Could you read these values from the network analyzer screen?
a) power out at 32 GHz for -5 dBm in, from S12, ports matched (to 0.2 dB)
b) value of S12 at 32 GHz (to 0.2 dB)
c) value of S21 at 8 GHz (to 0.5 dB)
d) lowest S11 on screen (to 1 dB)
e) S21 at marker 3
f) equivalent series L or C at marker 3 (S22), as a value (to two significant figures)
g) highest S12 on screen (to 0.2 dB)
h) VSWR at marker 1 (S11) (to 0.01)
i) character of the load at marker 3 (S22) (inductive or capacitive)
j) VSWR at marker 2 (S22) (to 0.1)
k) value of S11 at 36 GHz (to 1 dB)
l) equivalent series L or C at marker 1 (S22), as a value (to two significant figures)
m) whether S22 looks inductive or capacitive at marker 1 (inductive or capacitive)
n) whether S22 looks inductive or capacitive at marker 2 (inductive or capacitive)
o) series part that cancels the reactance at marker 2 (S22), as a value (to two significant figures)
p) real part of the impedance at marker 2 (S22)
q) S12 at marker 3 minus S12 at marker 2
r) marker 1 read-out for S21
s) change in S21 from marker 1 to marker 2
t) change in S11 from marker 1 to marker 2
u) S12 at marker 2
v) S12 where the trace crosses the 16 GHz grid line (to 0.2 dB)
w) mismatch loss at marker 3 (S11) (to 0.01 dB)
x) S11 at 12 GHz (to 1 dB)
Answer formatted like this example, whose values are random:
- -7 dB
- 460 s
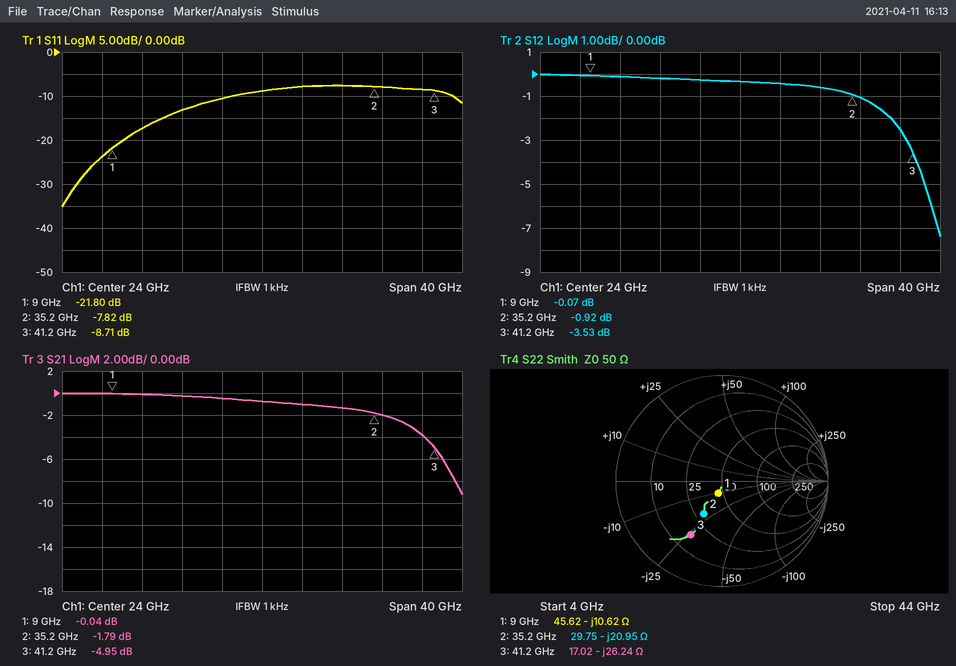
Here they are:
- -5.6 dBm
- -0.6 dB
- 0.0 dB
- -35 dB
- -4.95 dB
- 150 fF
- 0.0 dB
- 1.18
- capacitive
- 2.1
- -8 dB
- 1.7 pF
- capacitive
- capacitive
- 95 pH
- 29.75 Ω
- -2.61 dB
- -0.04 dB
- -1.75 dB
- 13.98 dB
- -0.92 dB
- -0.2 dB
- 0.63 dB
- -17 dB
